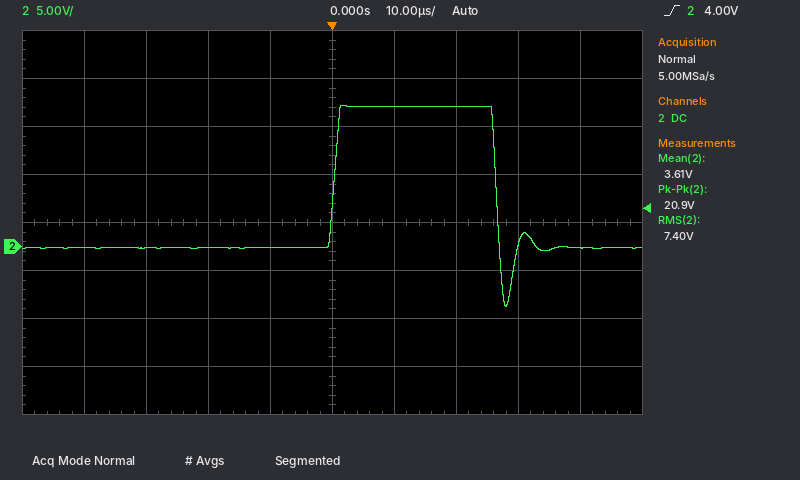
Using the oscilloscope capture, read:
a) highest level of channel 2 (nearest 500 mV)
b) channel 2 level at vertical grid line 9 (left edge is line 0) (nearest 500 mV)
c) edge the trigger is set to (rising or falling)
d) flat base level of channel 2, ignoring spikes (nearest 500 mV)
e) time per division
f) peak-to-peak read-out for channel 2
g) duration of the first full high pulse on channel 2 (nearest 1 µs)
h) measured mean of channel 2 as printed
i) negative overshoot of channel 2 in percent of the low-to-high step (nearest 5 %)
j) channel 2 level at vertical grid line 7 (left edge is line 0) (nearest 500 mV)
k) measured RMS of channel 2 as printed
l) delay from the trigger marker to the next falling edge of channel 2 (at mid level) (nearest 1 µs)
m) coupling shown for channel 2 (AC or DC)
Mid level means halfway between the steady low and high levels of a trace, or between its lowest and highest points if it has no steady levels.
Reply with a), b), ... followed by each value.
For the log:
a) 14.5 V
b) 0.0 V
c) rising
d) 0.0 V
e) 10 µs
f) 20.9 V
g) 26 µs
h) 3.61 V
i) 40 %
j) 14.5 V
k) 7.40 V
l) 26 µs
m) DC
